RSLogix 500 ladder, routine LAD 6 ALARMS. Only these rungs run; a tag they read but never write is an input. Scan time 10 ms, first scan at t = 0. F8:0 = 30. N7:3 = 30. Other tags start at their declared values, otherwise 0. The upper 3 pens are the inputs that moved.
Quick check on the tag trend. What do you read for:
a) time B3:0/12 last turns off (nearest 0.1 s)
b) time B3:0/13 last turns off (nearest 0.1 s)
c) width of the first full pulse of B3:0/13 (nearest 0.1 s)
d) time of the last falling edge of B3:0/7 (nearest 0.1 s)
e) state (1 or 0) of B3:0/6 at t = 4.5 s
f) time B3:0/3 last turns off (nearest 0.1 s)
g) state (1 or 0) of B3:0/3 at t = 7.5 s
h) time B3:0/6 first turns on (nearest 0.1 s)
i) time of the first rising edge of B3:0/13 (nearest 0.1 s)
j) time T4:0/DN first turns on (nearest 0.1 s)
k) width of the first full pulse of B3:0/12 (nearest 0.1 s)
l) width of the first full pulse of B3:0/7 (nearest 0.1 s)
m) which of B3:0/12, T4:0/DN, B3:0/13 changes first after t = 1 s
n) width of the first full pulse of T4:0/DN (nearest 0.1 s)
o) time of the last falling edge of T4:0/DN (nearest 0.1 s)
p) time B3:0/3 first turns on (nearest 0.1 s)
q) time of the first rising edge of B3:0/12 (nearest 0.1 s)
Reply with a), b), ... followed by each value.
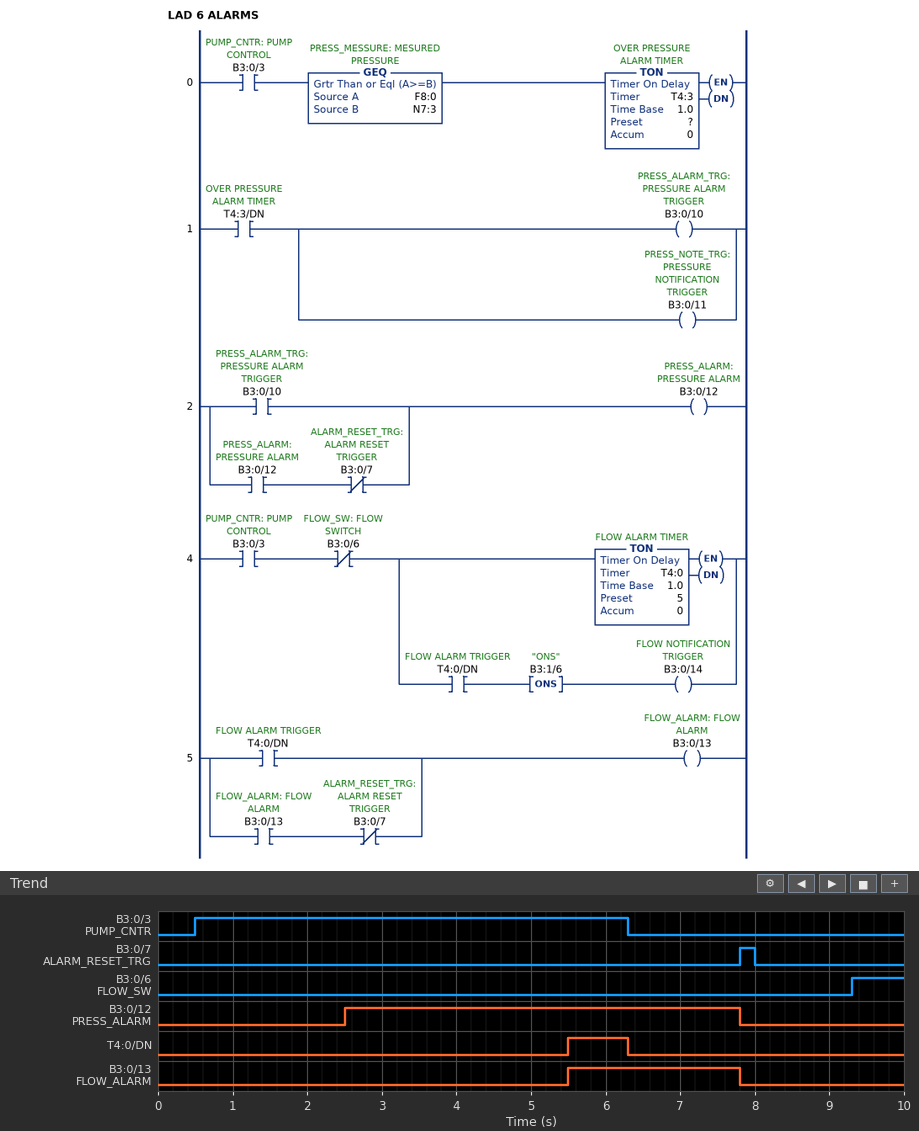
a) 7.8 s
b) 7.8 s
c) 2.3 s
d) 8.0 s
e) 0
f) 6.3 s
g) 0
h) 9.3 s
i) 5.5 s
j) 5.5 s
k) 5.3 s
l) 0.2 s
m) B3:0/12
n) 0.8 s
o) 6.3 s
p) 0.5 s
q) 2.5 s
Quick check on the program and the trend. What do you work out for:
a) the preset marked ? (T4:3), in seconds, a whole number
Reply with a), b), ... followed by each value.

a) 2 s
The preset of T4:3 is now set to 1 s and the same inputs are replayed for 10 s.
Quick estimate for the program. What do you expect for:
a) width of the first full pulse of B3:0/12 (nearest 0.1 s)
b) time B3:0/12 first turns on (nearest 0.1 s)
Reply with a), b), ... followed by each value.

a) 6.3 s
b) 1.5 s
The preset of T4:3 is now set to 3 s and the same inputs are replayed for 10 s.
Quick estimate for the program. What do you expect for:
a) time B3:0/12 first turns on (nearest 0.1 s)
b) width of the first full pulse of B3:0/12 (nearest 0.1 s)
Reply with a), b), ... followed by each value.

a) 3.5 s
b) 4.3 s
